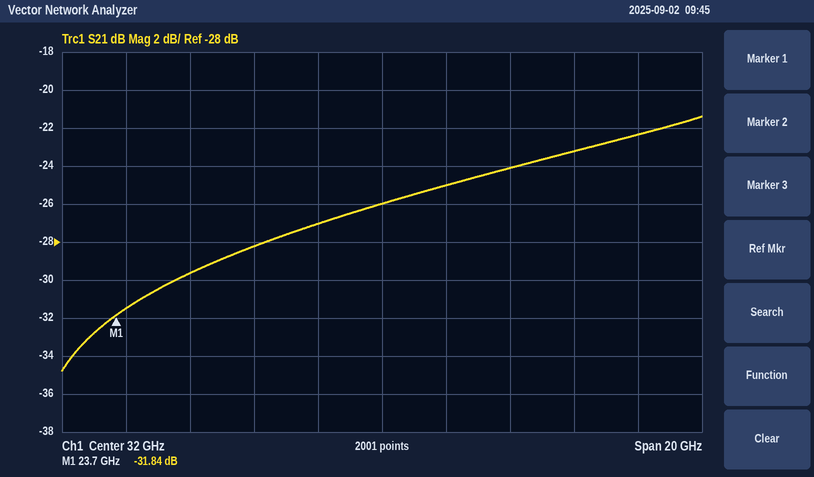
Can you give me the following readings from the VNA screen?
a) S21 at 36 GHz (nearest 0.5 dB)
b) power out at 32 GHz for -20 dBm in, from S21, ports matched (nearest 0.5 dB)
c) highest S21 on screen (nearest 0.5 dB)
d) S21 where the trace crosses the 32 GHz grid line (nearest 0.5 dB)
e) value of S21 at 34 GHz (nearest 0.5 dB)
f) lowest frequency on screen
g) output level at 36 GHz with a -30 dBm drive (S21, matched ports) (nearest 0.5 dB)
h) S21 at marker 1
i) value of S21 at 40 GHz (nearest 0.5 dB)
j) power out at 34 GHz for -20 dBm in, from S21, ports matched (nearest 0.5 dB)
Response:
-24.0 dB
-46.0 dBm
-21.5 dB
-26.0 dB
-25.0 dB
22 GHz
-54.0 dBm
-31.84 dB
-22.5 dB
-45.0 dBm
